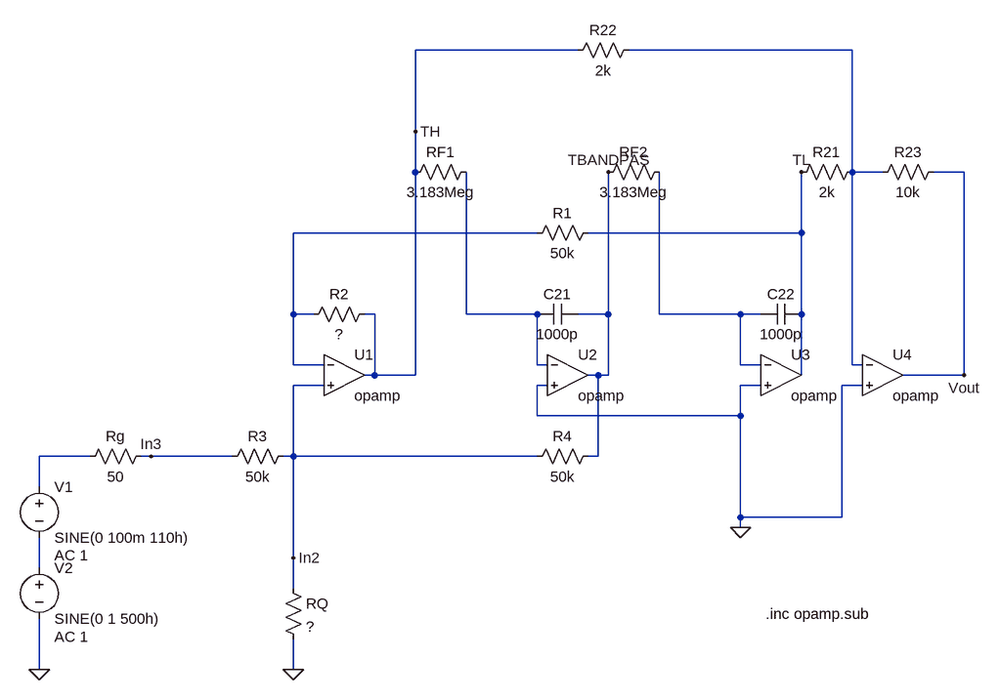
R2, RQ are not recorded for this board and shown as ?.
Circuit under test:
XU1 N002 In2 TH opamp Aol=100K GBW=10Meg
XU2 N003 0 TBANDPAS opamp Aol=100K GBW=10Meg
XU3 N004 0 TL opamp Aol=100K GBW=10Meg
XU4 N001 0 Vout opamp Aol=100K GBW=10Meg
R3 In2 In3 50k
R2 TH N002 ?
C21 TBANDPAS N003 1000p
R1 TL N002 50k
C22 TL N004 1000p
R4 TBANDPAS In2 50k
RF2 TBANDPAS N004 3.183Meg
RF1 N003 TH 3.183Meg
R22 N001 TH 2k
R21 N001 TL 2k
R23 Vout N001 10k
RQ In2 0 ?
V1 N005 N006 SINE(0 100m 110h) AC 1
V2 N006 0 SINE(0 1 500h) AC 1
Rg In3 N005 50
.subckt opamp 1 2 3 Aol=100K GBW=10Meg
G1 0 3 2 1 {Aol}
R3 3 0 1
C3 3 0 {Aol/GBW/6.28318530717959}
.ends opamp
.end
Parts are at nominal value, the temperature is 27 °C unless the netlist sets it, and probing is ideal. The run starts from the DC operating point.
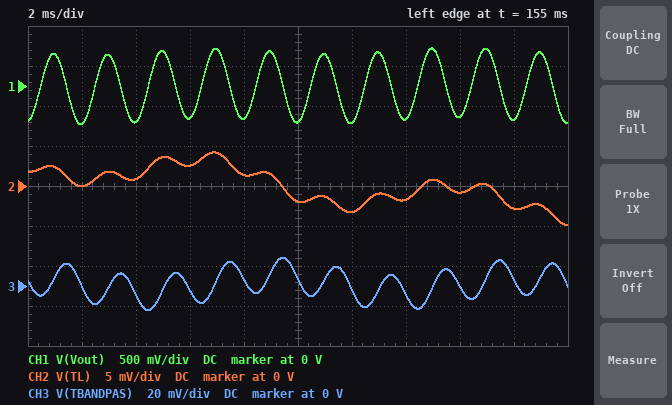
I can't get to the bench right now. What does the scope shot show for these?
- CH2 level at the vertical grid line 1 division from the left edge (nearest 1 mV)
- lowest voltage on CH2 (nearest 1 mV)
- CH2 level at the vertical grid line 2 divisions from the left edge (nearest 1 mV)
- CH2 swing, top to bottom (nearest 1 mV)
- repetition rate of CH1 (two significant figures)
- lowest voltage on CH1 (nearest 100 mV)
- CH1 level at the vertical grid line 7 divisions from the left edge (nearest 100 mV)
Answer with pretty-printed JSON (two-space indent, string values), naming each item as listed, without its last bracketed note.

{
  "CH2 level at the vertical grid line 1 division from the left edge": "0 V",
  "lowest voltage on CH2": "-5 mV",
  "CH2 level at the vertical grid line 2 divisions from the left edge": "1 mV",
  "CH2 swing, top to bottom": "9 mV",
  "repetition rate of CH1": "500 Hz",
  "lowest voltage on CH1": "-500 mV",
  "CH1 level at the vertical grid line 7 divisions from the left edge": "-400 mV"
}
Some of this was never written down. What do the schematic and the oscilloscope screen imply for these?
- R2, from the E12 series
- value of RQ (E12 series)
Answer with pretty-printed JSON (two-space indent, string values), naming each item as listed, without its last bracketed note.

{
  "R2, from the E12 series": "15 kΩ",
  "value of RQ": "3.9 kΩ"
}
